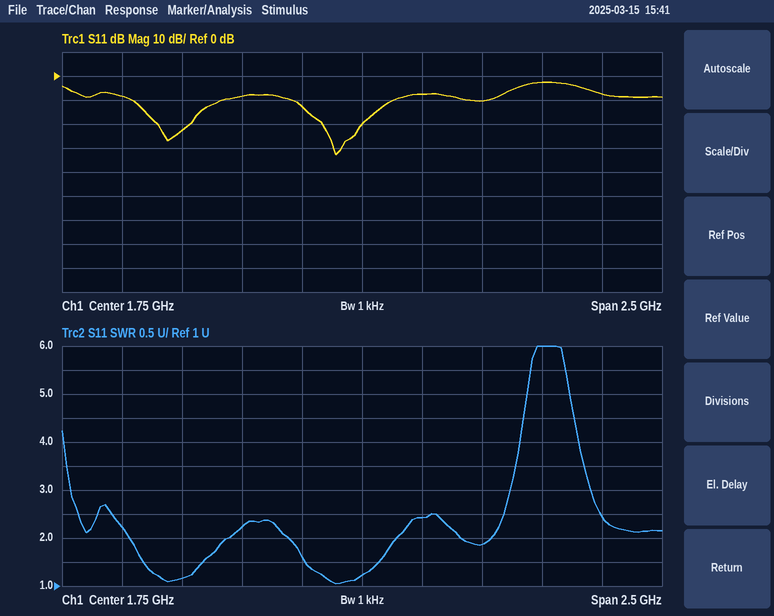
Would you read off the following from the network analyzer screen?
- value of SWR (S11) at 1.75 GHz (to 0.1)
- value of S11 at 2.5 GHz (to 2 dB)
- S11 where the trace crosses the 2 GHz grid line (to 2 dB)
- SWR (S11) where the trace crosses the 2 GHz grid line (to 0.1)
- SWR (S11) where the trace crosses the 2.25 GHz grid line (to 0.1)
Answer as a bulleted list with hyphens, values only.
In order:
- 1.2
- -2 dB
- -8 dB
- 2.4
- 1.9
